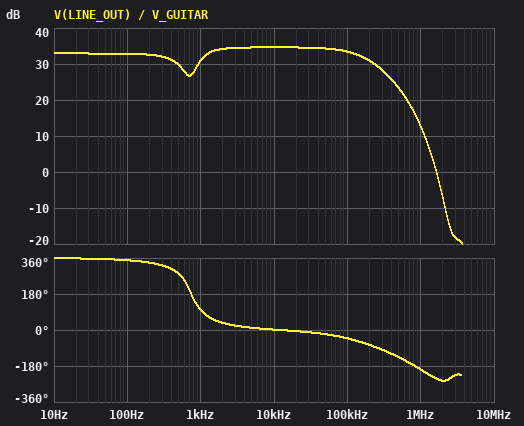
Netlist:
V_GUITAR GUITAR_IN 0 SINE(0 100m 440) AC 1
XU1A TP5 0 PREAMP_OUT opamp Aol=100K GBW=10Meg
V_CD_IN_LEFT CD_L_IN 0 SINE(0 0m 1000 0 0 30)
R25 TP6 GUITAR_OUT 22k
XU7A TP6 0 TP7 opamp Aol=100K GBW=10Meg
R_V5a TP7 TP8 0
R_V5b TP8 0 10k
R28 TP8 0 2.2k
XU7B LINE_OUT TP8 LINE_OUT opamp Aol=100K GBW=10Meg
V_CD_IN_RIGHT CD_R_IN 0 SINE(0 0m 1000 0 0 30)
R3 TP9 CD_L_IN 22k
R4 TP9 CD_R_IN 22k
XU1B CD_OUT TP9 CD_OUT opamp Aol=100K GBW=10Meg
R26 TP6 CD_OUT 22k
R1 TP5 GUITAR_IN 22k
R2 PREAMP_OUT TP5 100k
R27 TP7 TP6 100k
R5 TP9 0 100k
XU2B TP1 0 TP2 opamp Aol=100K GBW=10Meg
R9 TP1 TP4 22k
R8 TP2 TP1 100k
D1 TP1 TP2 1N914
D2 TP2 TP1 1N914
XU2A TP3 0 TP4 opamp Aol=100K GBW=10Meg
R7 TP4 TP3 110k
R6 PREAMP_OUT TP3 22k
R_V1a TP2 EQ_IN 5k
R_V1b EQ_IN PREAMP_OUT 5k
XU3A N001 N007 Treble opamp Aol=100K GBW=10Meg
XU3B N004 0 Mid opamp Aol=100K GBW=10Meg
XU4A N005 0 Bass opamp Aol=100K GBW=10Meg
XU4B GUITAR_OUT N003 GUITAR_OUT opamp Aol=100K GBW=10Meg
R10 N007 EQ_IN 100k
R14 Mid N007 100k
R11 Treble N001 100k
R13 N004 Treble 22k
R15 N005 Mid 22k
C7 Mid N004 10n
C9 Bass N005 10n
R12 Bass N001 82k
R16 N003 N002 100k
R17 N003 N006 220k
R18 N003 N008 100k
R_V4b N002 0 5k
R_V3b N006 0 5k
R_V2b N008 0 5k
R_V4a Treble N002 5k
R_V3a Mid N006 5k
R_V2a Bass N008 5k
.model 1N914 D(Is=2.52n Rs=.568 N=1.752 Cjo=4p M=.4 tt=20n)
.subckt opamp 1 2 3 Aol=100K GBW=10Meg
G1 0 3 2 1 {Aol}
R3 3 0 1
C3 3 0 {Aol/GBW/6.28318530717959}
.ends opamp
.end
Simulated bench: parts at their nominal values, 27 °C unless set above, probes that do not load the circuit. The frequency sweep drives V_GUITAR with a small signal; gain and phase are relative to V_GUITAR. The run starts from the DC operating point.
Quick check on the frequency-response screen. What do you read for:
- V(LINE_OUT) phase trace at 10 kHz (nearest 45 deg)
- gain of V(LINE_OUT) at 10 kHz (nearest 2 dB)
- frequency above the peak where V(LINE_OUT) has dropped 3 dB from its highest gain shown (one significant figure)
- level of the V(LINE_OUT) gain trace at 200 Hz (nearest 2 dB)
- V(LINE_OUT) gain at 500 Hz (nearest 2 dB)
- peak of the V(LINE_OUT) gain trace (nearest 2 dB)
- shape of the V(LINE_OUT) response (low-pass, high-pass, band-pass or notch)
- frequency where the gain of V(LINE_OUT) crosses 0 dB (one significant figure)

0 deg
34 dB
200 kHz
32 dB
30 dB
34 dB
low-pass
2 MHz
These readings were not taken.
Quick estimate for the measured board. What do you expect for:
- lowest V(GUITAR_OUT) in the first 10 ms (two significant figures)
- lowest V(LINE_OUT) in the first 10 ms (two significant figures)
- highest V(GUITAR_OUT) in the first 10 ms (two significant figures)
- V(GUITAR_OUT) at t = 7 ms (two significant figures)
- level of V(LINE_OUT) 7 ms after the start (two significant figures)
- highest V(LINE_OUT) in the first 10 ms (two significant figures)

-84 mV
-380 mV
84 mV
41 mV
-190 mV
380 mV
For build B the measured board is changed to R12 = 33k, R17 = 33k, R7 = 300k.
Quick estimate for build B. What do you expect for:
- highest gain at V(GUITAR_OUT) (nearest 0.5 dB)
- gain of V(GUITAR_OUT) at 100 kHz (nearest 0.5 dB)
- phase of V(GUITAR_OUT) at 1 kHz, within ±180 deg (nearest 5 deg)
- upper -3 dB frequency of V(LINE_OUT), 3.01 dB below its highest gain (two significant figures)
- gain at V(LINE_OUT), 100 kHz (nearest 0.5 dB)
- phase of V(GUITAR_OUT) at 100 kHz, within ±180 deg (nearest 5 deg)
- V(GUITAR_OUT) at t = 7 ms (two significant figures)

33.0 dB
28.0 dB
10 deg
4.6 kHz
41.0 dB
140 deg
110 mV
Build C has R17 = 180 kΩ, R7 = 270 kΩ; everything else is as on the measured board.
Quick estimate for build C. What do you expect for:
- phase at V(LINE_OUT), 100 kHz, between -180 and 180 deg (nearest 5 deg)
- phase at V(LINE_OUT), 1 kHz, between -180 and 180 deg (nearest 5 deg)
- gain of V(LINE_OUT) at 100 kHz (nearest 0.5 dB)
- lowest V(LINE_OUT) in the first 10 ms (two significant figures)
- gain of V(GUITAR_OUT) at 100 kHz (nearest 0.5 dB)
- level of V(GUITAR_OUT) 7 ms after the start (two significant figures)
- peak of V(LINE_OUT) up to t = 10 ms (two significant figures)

-45 deg
105 deg
40.5 dB
-400 mV
27.5 dB
49 mV
400 mV
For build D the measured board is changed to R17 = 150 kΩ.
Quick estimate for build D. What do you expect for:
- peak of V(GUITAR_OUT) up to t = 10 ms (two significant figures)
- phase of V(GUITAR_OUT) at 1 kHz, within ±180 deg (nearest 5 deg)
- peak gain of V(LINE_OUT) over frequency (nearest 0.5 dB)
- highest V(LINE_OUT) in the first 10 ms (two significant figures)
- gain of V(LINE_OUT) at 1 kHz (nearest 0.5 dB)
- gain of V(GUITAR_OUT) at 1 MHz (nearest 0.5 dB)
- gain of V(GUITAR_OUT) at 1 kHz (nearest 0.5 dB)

81 mV
-70 deg
34.0 dB
370 mV
31.5 dB
2.0 dB
18.5 dB
